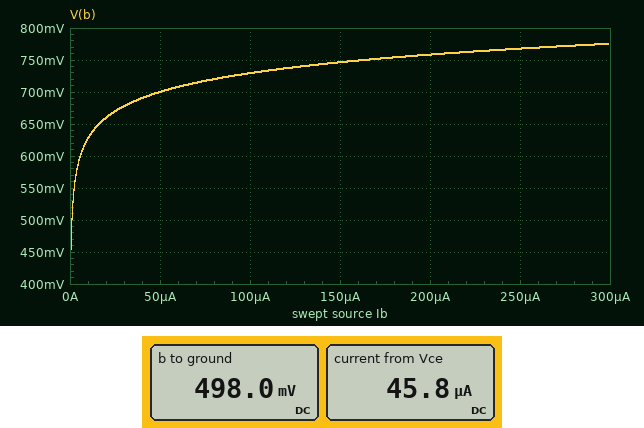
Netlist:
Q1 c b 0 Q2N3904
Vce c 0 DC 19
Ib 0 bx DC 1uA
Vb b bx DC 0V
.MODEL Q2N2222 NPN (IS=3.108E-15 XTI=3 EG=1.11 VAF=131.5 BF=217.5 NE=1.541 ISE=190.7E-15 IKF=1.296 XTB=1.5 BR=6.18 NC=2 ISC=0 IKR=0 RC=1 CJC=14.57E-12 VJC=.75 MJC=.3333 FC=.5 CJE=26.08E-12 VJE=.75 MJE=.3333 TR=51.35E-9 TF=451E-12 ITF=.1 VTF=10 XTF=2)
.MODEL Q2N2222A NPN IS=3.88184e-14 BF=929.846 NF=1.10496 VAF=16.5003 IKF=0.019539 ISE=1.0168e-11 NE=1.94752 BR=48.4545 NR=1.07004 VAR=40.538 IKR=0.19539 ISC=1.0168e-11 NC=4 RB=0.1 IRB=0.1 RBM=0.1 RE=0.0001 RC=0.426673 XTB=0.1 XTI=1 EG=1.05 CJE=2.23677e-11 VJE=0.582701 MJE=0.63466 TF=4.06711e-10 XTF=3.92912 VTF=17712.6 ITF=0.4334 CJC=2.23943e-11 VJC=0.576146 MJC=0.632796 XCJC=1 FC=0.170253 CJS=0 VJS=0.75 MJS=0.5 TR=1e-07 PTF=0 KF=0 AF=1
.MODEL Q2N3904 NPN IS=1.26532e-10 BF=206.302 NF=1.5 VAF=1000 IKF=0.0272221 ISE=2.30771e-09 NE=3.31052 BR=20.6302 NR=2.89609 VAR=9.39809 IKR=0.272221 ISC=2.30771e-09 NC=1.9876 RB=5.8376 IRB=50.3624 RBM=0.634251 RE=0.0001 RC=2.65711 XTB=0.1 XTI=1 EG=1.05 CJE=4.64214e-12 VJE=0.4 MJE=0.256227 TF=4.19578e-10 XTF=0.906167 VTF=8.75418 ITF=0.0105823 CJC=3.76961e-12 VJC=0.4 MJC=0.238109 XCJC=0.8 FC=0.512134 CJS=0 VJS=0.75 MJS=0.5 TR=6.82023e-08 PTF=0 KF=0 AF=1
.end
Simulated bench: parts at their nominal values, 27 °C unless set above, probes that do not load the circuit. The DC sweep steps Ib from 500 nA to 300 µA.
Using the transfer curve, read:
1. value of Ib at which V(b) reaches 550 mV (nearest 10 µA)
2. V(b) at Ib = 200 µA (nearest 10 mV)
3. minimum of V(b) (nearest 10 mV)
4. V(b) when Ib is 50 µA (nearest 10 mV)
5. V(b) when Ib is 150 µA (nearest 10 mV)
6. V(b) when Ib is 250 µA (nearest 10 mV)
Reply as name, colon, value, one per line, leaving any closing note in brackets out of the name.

value of Ib at which V(b) reaches 550 mV: 0 A
V(b) at Ib = 200 µA: 760 mV
minimum of V(b): 450 mV
V(b) when Ib is 50 µA: 700 mV
V(b) when Ib is 150 µA: 750 mV
V(b) when Ib is 250 µA: 770 mV
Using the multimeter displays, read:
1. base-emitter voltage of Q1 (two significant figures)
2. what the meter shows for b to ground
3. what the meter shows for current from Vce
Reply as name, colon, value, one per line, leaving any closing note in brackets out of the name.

base-emitter voltage of Q1: 500 mV
what the meter shows for b to ground: 498.0 mV
what the meter shows for current from Vce: 45.8 µA
